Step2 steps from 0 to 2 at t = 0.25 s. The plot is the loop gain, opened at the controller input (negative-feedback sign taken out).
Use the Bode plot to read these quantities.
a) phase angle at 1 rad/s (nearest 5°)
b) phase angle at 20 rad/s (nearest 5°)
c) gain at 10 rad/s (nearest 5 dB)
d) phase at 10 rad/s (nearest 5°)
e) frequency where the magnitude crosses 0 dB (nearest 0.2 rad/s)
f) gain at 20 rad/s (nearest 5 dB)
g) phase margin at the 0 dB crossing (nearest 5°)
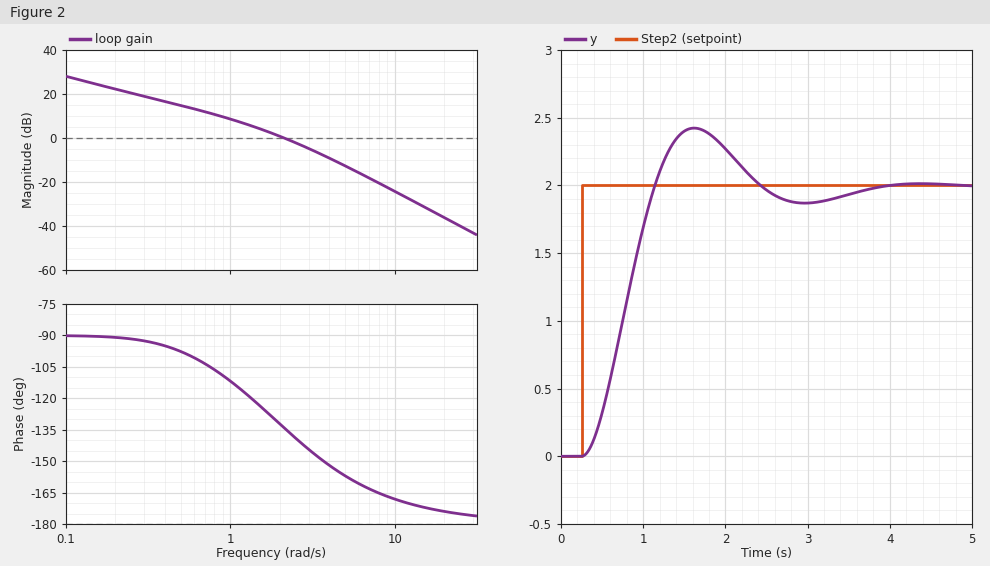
-110°
-175°
-25 dB
-170°
2.2 rad/s
-35 dB
45°
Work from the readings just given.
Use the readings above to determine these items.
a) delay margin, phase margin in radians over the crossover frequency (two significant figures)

0.36 s
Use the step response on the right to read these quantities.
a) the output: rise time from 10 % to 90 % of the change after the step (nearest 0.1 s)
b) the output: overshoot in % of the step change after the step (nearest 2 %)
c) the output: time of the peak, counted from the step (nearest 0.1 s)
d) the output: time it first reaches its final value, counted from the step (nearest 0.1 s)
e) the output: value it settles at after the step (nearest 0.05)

0.6 s
22 %
1.4 s
0.9 s
2.00
